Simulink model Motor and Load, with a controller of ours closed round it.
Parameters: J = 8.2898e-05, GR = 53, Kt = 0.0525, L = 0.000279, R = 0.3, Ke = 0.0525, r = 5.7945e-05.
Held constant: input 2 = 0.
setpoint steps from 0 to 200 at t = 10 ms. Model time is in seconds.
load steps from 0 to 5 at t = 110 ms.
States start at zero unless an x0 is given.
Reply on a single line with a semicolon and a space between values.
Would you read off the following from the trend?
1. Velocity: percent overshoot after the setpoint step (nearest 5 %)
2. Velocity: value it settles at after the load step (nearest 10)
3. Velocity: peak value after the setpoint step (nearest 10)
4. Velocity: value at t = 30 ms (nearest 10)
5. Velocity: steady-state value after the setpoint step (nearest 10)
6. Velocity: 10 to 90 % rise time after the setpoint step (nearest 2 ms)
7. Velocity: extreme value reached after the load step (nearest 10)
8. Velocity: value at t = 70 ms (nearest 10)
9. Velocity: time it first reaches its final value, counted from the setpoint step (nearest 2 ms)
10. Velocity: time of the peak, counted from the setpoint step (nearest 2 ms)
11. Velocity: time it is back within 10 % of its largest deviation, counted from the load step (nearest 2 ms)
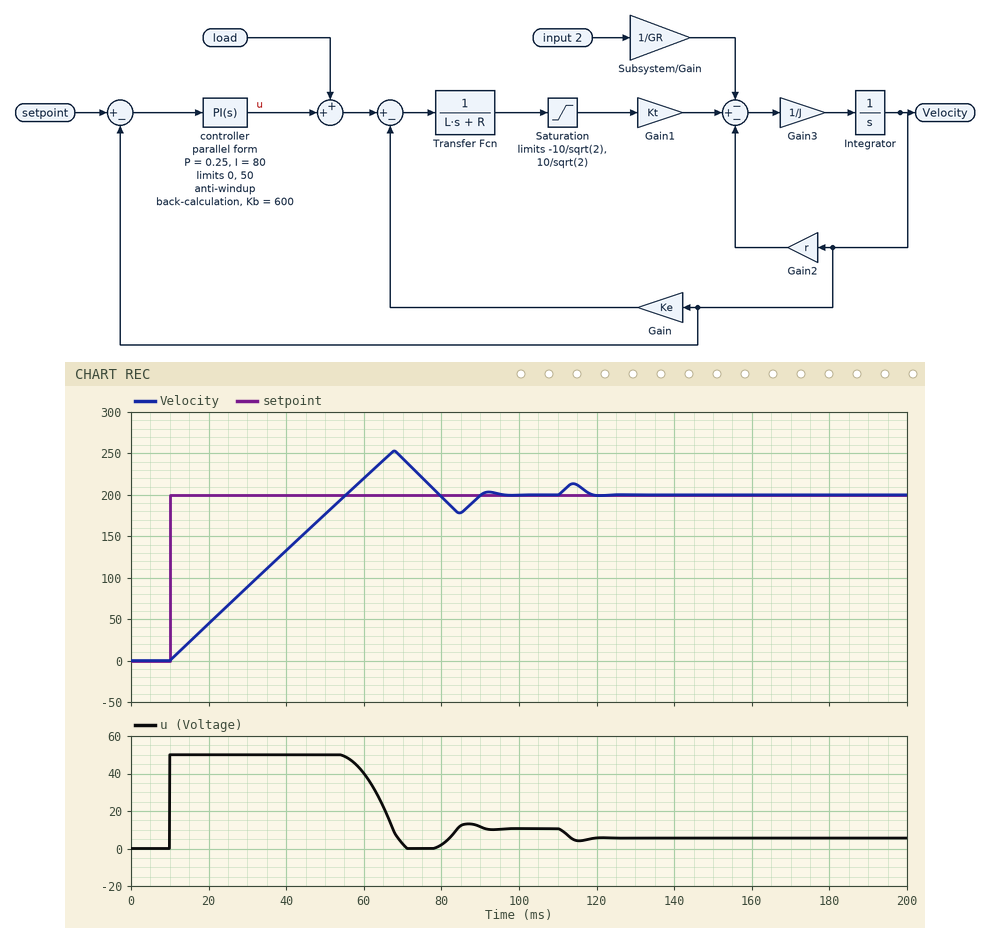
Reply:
25 %; 200; 250; 90; 200; 36 ms; 210; 240; 46 ms; 58 ms; 8 ms
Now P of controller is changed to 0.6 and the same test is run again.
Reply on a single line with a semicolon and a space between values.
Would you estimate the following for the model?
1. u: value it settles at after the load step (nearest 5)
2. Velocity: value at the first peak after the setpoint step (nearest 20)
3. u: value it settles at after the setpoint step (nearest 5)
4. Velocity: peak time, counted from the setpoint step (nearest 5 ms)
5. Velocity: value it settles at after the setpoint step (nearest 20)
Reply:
5; 240; 10; 55 ms; 200
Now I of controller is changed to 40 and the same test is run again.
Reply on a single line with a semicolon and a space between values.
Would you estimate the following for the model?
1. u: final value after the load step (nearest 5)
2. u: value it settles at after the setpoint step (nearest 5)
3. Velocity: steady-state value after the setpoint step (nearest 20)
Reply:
5; 10; 200
